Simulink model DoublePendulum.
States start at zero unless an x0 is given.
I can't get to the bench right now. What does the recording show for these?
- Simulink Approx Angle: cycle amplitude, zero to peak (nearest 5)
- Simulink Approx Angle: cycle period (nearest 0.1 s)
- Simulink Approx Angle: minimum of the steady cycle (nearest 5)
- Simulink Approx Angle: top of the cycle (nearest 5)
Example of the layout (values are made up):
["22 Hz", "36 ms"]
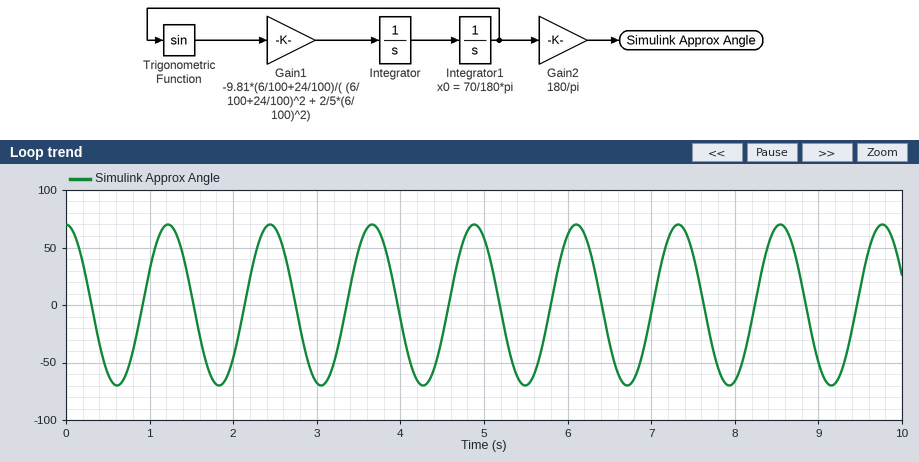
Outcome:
["70", "1.2 s", "-70", "70"]
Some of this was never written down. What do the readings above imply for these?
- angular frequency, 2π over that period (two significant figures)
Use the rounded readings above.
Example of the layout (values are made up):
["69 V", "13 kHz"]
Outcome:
["5.2 rad/s"]
